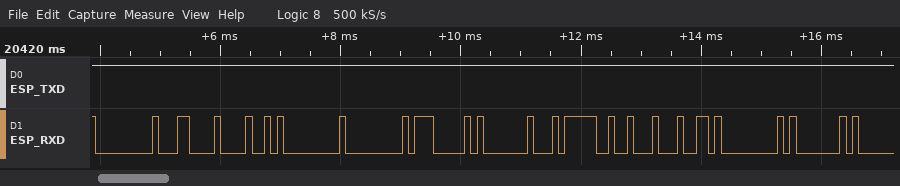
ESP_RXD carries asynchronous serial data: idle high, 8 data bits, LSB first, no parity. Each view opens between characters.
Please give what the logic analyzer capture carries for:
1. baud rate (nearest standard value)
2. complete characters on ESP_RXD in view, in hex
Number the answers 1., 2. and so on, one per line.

1. 9600 baud
2. 00, 0C, 48, 00, 00, 07, 01, F4, 12, 64, 00, 01
